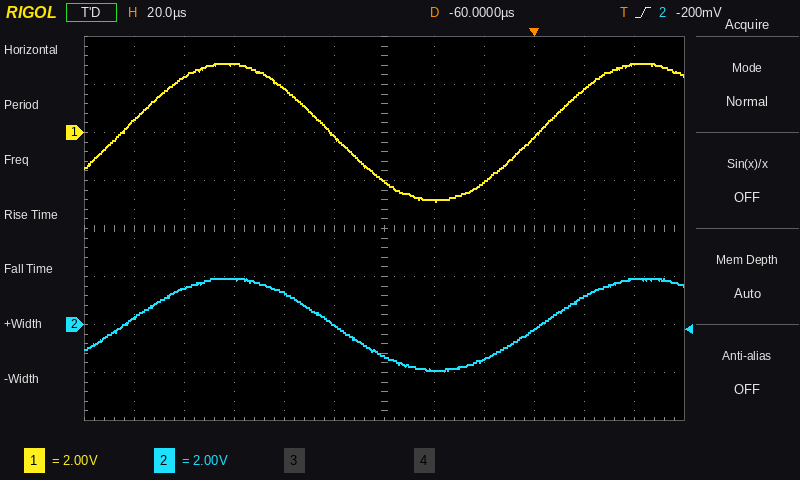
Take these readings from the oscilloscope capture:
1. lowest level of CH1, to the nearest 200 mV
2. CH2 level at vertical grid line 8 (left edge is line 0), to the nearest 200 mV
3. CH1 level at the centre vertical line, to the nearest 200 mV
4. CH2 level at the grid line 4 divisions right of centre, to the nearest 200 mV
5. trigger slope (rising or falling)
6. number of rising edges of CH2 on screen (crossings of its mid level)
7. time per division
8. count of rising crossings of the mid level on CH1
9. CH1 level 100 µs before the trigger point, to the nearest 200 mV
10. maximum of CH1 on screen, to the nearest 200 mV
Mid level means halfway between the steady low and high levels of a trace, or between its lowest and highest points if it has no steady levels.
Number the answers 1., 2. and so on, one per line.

1. -2.8 V
2. -1.4 V
3. -2.0 V
4. 1.2 V
5. rising
6. 2
7. 20 µs
8. 2
9. 1.8 V
10. 2.8 V
